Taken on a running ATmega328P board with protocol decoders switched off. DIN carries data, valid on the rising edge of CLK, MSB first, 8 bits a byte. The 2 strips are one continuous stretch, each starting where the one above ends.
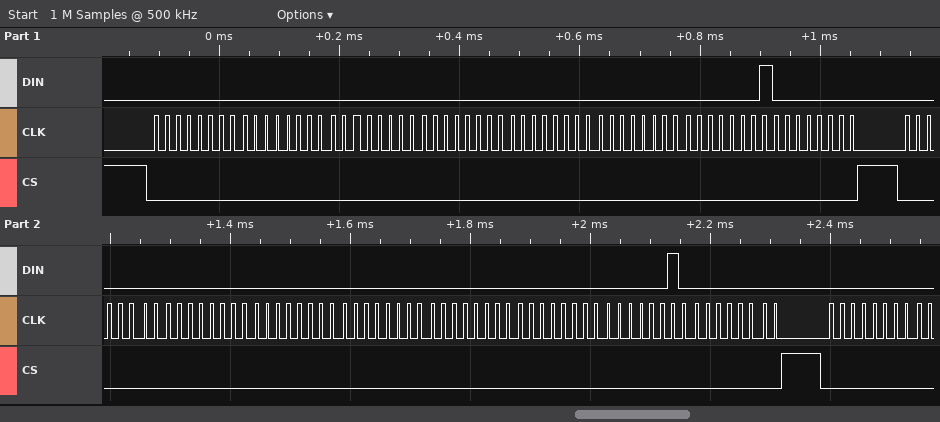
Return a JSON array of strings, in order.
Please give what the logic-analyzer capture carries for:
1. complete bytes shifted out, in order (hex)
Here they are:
["00 00 00 00 00 00 01 00 00 00 00 00 00 00 02 00 00"]
